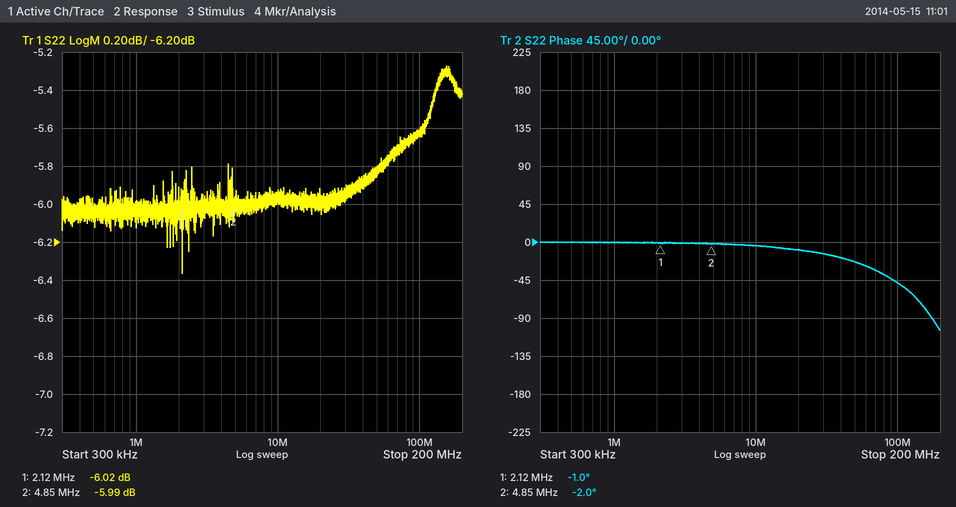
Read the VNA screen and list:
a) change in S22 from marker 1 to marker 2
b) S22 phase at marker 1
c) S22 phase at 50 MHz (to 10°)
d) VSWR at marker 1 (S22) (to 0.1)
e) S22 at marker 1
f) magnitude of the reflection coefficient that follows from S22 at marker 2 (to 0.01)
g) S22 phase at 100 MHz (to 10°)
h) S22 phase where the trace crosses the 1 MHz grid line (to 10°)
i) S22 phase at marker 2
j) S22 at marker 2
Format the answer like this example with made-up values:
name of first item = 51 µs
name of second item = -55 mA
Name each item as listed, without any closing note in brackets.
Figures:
change in S22 from marker 1 to marker 2 = 0.03 dB
S22 phase at marker 1 = -1.0°
S22 phase at 50 MHz = -20°
VSWR at marker 1 (S22) = 3.0
S22 at marker 1 = -6.02 dB
magnitude of the reflection coefficient that follows from S22 at marker 2 = 0.50
S22 phase at 100 MHz = -50°
S22 phase where the trace crosses the 1 MHz grid line = 0°
S22 phase at marker 2 = -2.0°
S22 at marker 2 = -5.99 dB
